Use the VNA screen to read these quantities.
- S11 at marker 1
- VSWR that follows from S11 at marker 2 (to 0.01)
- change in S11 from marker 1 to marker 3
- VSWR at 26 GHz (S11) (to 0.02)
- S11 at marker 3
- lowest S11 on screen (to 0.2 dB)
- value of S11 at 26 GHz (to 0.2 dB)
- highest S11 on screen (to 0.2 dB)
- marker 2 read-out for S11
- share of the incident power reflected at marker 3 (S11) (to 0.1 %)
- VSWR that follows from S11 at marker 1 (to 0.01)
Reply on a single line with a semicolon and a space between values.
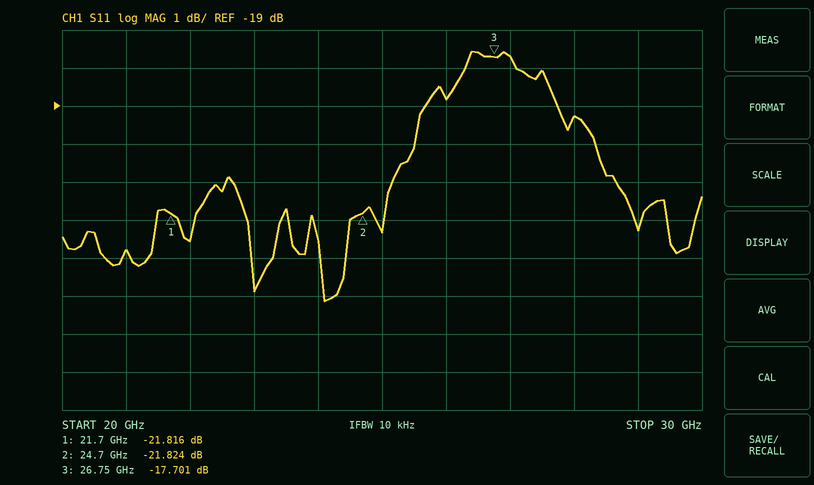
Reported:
-21.816 dB; 1.18; 4.115 dB; 1.26; -17.701 dB; -24.2 dB; -18.8 dB; -17.6 dB; -21.824 dB; 1.7 %; 1.18
